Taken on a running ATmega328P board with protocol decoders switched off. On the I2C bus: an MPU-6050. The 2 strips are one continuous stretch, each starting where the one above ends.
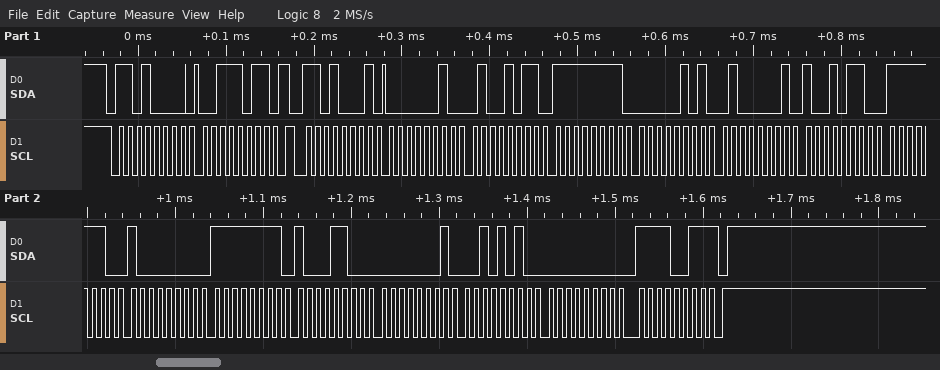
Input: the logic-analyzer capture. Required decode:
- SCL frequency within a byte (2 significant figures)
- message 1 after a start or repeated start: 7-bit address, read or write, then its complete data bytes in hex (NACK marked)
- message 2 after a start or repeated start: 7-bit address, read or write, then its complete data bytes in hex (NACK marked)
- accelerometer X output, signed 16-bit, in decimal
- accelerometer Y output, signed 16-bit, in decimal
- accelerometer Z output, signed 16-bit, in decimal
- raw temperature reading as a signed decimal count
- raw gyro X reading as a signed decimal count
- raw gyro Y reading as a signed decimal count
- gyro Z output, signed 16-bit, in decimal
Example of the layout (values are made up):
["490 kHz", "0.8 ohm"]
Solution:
["100 kHz", "0x68 write: 3B", "0x68 read: 02 4B FF 05 41 96 FE 80 FF 8C 01 2A 00 F3 NACK", "587", "-251", "16790", "-384", "-116", "298", "243"]
